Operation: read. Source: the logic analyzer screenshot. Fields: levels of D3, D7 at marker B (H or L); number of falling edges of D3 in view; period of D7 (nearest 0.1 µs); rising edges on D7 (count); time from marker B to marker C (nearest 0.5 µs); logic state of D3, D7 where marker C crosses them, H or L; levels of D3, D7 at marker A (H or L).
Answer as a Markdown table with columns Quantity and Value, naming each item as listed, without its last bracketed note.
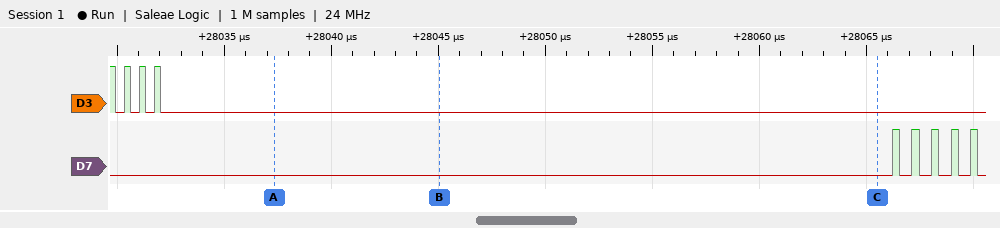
| Quantity | Value |
|---|---|
| levels of D3, D7 at marker B | D3=L, D7=L |
| number of falling edges of D3 in view | 4 |
| period of D7 | 0.9 µs |
| rising edges on D7 | 5 |
| time from marker B to marker C | 20.5 µs |
| logic state of D3, D7 where marker C crosses them, H or L | D3=L, D7=L |
| levels of D3, D7 at marker A | D3=L, D7=L |
